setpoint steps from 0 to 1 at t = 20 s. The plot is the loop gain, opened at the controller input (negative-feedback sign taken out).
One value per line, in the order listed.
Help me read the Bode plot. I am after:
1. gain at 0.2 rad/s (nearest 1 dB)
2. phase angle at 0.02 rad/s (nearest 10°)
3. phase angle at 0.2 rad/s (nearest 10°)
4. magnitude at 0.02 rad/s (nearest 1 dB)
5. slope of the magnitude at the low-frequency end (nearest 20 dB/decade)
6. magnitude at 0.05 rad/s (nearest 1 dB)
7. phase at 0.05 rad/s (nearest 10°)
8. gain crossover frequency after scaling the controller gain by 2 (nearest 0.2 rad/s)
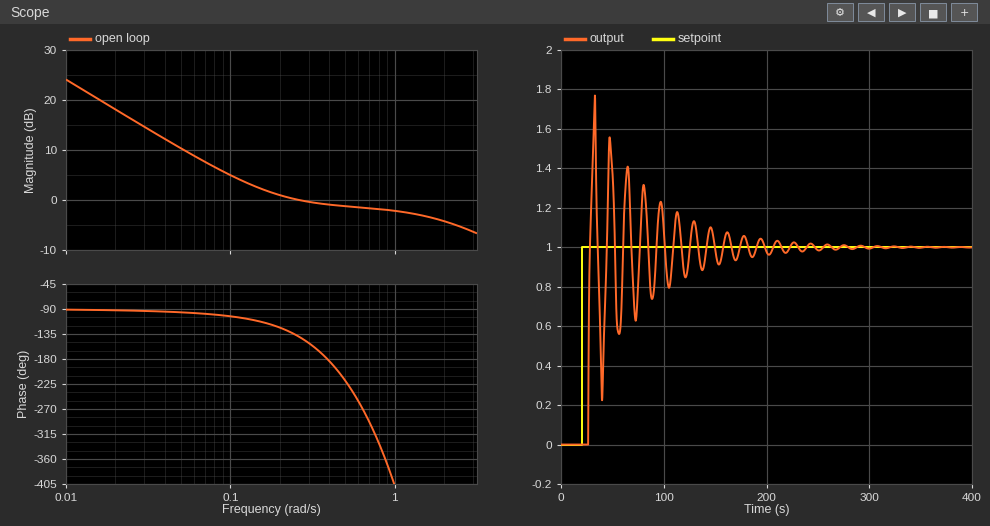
1 dB
-90°
-120°
18 dB
-20 dB/decade
10 dB
-100°
2.8 rad/s
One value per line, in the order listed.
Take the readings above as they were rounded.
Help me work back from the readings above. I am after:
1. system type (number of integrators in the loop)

1
